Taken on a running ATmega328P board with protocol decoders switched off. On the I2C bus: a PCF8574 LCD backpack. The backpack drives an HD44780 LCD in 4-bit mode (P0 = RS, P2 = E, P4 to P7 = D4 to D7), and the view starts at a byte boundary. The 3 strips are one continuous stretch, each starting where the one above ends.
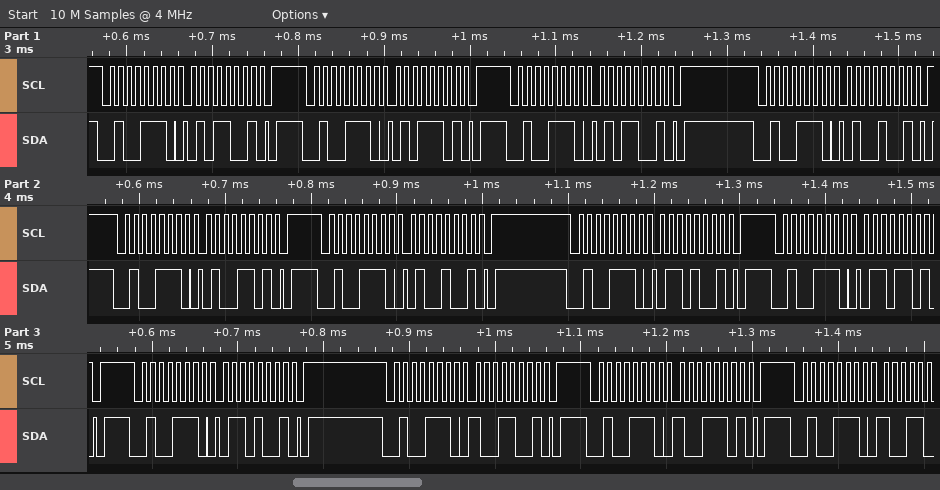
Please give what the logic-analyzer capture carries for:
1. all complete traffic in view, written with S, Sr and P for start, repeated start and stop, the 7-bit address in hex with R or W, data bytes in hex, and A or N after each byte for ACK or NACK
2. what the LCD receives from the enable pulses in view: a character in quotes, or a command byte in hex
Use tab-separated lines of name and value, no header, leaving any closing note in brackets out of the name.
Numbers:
all complete traffic in view, written with S, Sr and P for start, repeated start and stop, the 7-bit address in hex with R or W, data bytes in hex, and A or N after each byte for ACK or NACK	S 27W A 59 A P S 27W A 5D A P S 27W A 59 A P S 27W A 49 A P S 27W A 4D A P S 27W A 49 A P S 27W A 69 A P S 27W A 6D A P S 27W A 69 A P S 27W A 99 A P S 27W A 9D A P S 27W A
what the LCD receives from the enable pulses in view: a character in quotes, or a command byte in hex	'T'
